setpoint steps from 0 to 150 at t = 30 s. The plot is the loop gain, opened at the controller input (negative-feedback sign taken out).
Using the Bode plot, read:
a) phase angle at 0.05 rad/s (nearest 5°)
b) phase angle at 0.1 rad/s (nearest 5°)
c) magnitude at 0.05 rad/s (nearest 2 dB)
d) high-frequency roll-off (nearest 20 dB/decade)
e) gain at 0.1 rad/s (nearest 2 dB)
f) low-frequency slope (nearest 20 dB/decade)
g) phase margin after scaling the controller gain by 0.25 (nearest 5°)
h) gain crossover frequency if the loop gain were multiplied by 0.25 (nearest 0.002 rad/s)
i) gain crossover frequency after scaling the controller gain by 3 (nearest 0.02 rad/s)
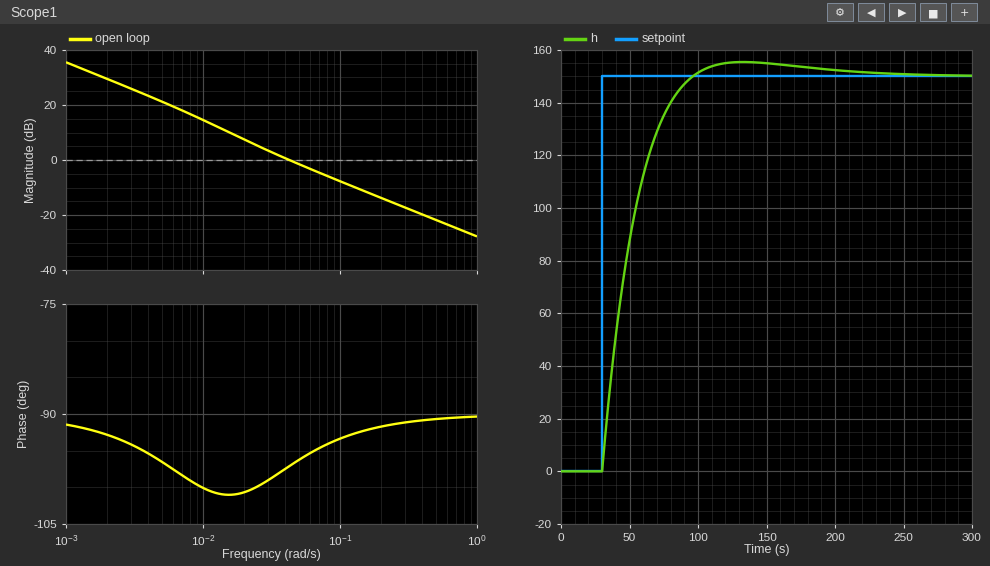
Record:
-95°
-95°
-2 dB
-20 dB/decade
-8 dB
-20 dB/decade
80°
0.012 rad/s
0.12 rad/s
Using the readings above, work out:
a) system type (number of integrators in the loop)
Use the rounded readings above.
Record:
1
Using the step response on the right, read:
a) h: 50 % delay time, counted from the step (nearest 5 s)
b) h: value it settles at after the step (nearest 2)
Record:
15 s
150
